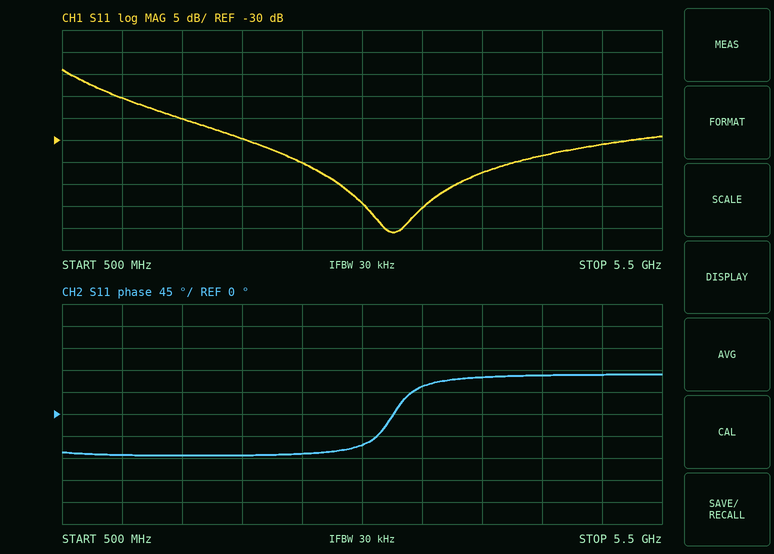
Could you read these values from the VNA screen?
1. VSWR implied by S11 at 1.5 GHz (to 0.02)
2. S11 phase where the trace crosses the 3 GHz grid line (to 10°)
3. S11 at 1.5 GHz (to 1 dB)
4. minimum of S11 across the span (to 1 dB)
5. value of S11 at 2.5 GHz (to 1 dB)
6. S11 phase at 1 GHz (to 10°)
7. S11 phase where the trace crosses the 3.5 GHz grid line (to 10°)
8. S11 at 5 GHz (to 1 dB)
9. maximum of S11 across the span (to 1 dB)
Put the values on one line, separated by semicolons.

1.12; -60°; -25 dB; -51 dB; -35 dB; -80°; 60°; -31 dB; -14 dB
